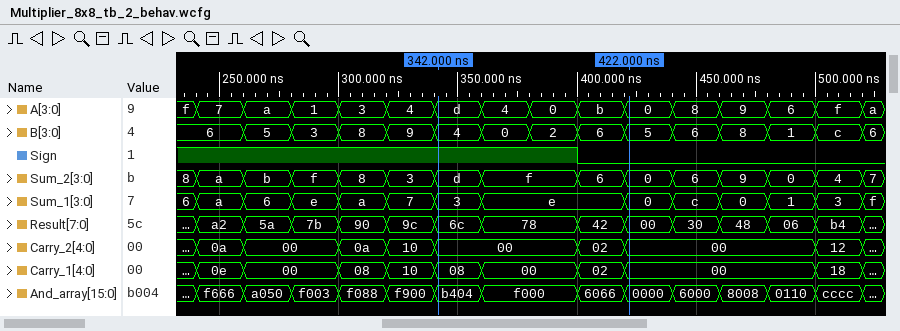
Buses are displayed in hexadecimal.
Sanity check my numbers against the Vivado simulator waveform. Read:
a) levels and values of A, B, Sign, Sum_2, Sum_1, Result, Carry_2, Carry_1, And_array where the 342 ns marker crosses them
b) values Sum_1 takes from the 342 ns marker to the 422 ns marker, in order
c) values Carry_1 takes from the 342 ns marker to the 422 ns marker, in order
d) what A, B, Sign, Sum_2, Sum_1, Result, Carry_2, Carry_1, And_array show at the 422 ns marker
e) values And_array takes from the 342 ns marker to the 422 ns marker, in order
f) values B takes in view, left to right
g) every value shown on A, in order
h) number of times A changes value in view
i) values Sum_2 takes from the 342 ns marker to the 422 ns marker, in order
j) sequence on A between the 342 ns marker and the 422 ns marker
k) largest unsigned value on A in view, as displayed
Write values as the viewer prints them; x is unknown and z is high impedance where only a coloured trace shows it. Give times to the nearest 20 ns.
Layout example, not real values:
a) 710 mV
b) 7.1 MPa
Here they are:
a) A=d, B=4, Sign=1, Sum_2=d, Sum_1=3, Result=6c, Carry_2=00, Carry_1=08, And_array=b404
b) 3, e, 0
c) 08, 00, 02, 00
d) A=0, B=5, Sign=0, Sum_2=0, Sum_1=0, Result=00, Carry_2=00, Carry_1=00, And_array=0000
e) b404, f000, 6066, 0000
f) 6, 5, 3, 8, 9, 4, 0, 2, 6, 5, 6, 8, 1, c, 6
g) f, 7, a, 1, 3, 4, d, 4, 0, b, 0, 8, 9, 6, f, a
h) 15
i) d, f, 6, 0
j) d, 4, 0, b, 0
k) f
